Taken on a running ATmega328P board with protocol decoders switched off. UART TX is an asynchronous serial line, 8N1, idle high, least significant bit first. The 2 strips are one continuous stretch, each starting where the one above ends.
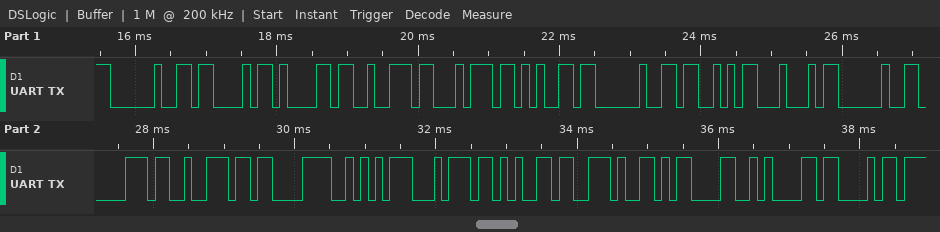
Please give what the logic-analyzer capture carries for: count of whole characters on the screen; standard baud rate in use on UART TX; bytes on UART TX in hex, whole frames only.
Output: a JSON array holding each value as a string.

["20", "9600 baud", "20 43 61 72 74 65 20 53 44 20 70 72 C3 AA 74 65 2E 0D 0A 43"]
